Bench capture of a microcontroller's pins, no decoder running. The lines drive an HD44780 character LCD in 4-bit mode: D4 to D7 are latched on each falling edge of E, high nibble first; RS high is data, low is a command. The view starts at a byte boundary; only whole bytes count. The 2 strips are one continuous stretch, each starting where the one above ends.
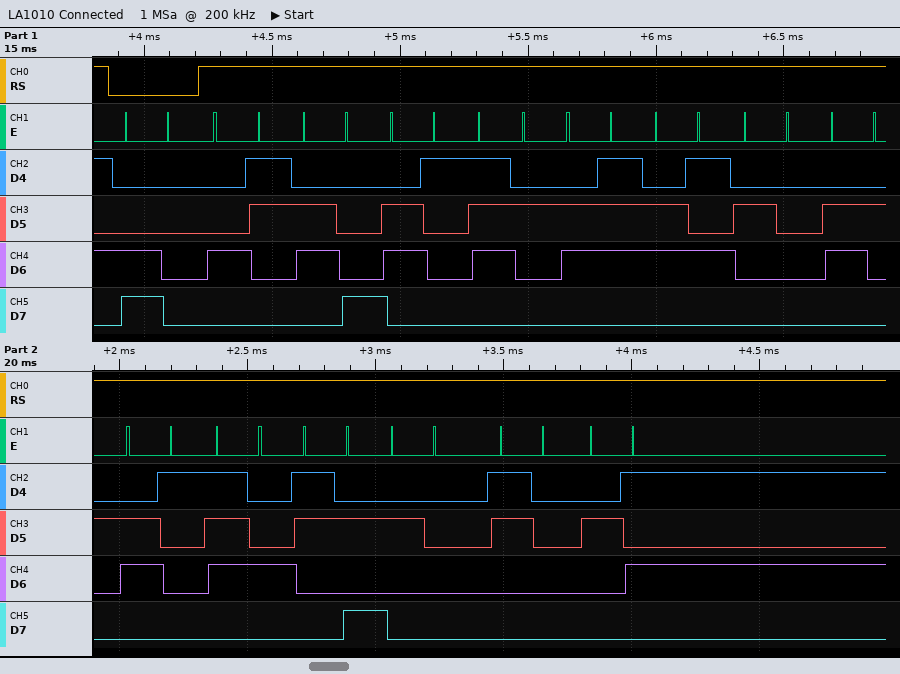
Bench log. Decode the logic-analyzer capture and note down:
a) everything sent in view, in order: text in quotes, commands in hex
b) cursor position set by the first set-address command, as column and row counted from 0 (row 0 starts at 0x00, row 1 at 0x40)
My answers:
0xC0 "Charge bat: 0%"
column 0, row 1
